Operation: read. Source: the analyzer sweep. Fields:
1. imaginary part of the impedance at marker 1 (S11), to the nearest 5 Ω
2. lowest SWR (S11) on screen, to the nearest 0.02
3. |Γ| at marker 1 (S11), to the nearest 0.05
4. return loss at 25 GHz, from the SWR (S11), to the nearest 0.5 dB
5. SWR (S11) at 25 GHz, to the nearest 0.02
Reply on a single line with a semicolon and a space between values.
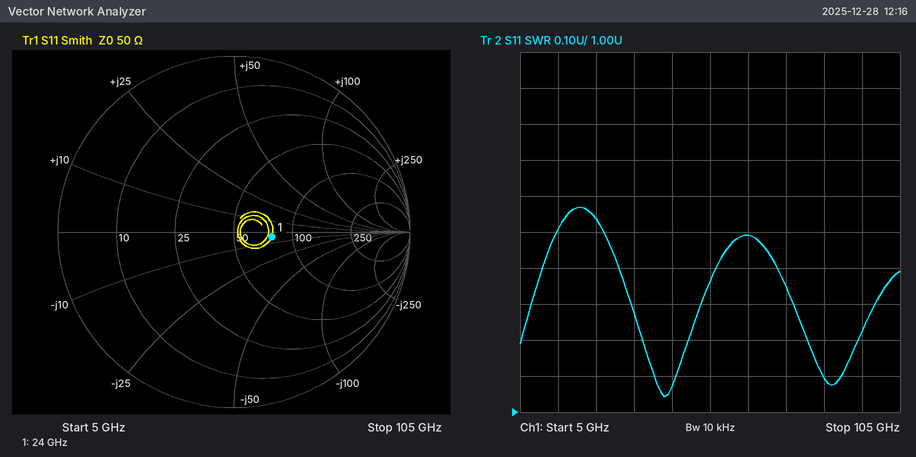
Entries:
-5 Ω; 1.04; 0.20; 13.5 dB; 1.54
